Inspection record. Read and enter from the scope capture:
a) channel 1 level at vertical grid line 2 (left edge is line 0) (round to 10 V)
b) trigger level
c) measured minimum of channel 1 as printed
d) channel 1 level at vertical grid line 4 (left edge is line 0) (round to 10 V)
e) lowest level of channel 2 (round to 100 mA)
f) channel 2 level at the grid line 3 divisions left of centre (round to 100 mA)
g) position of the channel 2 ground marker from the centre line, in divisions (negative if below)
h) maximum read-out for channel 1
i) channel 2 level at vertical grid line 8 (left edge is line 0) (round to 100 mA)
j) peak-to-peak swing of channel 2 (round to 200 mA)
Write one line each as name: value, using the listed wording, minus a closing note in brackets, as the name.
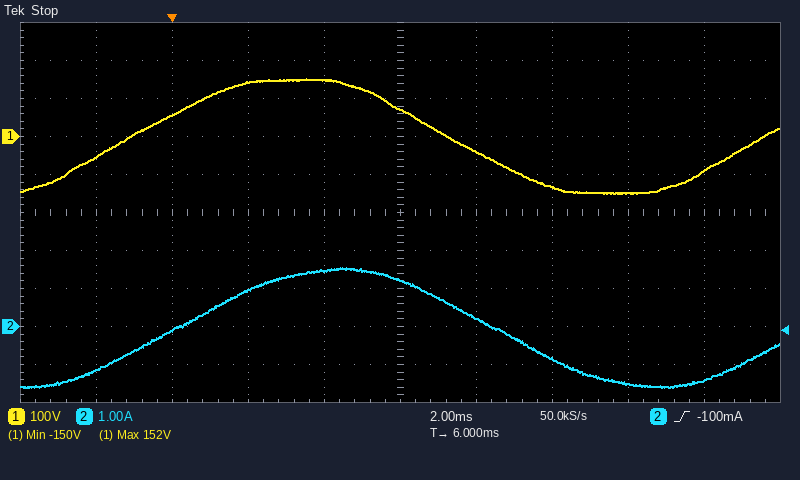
channel 1 level at vertical grid line 2 (left edge is line 0): 60 V
trigger level: -100 mA
measured minimum of channel 1 as printed: -150 V
channel 1 level at vertical grid line 4 (left edge is line 0): 150 V
lowest level of channel 2: -1.6 A
channel 2 level at the grid line 3 divisions left of centre: -100 mA
position of the channel 2 ground marker from the centre line, in divisions: -3.0 div
maximum read-out for channel 1: 152 V
channel 2 level at vertical grid line 8 (left edge is line 0): -1.5 A
peak-to-peak swing of channel 2: 3.2 A
